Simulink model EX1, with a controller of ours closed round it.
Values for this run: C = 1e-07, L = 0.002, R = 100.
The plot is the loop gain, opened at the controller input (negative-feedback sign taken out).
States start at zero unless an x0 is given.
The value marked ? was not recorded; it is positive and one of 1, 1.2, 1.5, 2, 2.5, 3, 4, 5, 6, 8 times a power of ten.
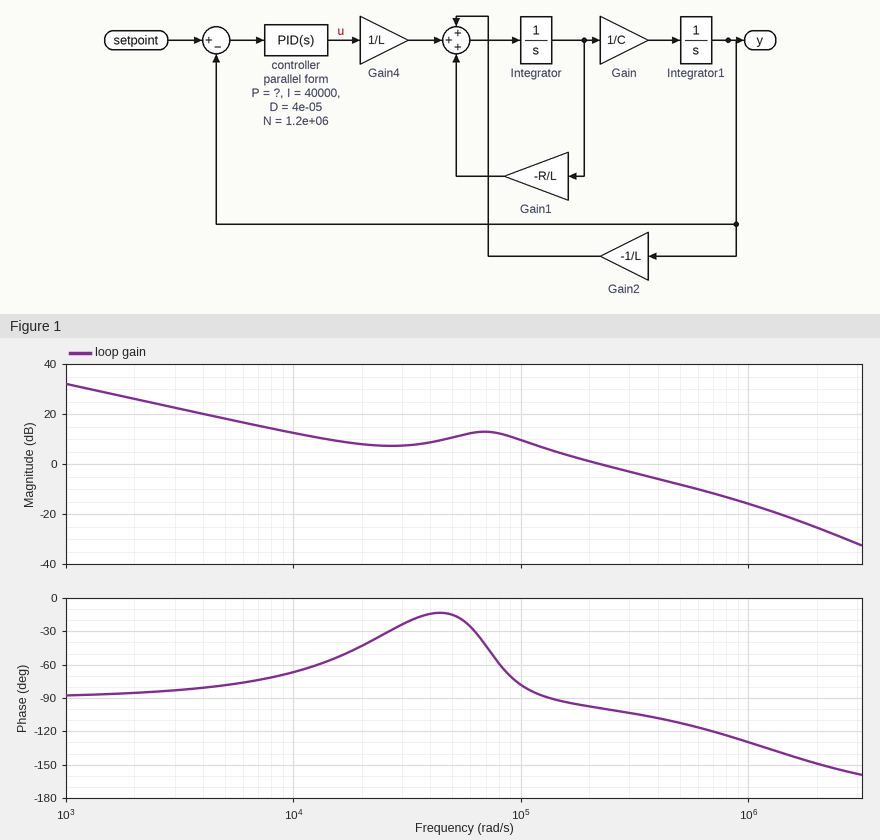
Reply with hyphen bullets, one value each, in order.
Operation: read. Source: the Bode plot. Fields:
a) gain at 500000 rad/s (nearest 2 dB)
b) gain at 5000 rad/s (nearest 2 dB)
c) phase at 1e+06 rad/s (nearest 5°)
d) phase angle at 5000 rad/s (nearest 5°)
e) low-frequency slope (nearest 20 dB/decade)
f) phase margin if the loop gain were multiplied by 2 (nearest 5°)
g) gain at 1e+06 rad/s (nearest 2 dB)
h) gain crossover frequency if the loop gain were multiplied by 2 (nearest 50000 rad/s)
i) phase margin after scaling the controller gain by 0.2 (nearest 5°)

- -8 dB
- 18 dB
- -130°
- -80°
- -20 dB/decade
- 70°
- -16 dB
- 400000 rad/s
- 110°
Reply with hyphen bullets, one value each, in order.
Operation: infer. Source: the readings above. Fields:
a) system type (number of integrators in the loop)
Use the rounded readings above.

- 1
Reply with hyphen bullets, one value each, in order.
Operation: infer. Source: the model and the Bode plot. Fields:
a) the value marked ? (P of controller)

- 2
